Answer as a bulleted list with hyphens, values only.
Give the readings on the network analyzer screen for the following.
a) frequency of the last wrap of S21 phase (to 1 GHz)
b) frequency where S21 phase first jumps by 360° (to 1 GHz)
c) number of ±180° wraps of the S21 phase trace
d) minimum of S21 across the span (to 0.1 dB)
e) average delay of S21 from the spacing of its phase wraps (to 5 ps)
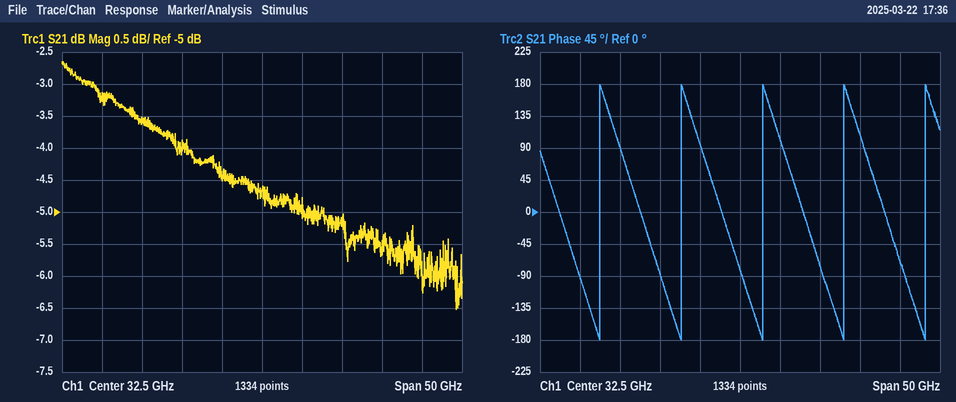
- 56 GHz
- 15 GHz
- 5
- -6.5 dB
- 100 ps
